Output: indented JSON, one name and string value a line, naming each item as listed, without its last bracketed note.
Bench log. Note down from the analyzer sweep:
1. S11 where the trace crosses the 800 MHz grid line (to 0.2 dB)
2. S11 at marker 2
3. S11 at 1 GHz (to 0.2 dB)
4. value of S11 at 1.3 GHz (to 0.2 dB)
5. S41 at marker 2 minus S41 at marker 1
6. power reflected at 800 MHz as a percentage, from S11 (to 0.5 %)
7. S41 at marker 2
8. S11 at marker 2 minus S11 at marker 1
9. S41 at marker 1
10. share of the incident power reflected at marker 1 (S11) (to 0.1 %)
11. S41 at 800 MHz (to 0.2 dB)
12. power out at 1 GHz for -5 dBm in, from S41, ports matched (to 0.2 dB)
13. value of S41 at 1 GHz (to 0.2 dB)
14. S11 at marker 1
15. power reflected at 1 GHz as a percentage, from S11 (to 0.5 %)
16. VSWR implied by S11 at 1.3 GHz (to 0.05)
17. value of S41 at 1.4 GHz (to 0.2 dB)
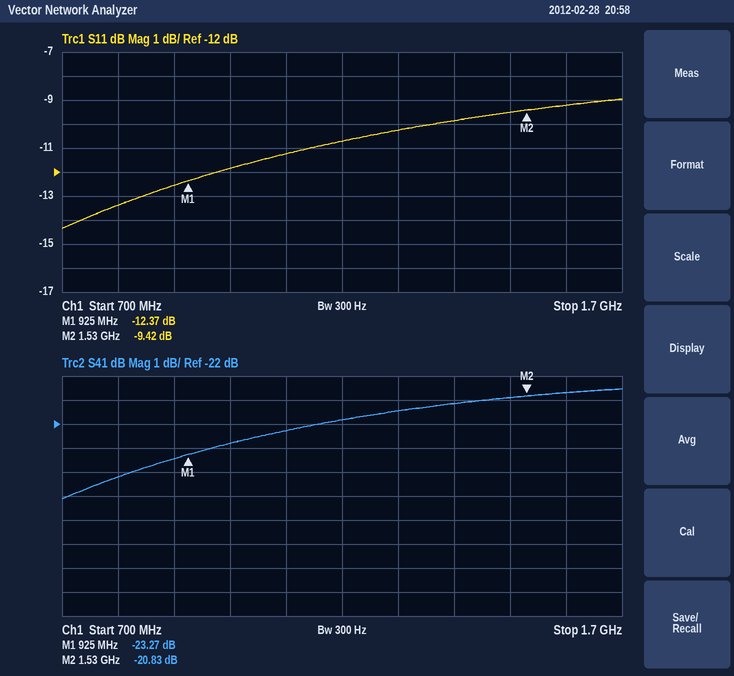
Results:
{
  "S11 where the trace crosses the 800 MHz grid line": "-13.4 dB",
  "S11 at marker 2": "-9.42 dB",
  "S11 at 1 GHz": "-11.8 dB",
  "value of S11 at 1.3 GHz": "-10.2 dB",
  "S41 at marker 2 minus S41 at marker 1": "2.44 dB",
  "power reflected at 800 MHz as a percentage, from S11": "4.5 %",
  "S41 at marker 2": "-20.83 dB",
  "S11 at marker 2 minus S11 at marker 1": "2.95 dB",
  "S41 at marker 1": "-23.27 dB",
  "share of the incident power reflected at marker 1 (S11)": "5.8 %",
  "S41 at 800 MHz": "-24.2 dB",
  "power out at 1 GHz for -5 dBm in, from S41, ports matched": "-27.8 dBm",
  "value of S41 at 1 GHz": "-22.8 dB",
  "S11 at marker 1": "-12.37 dB",
  "power reflected at 1 GHz as a percentage, from S11": "6.5 %",
  "VSWR implied by S11 at 1.3 GHz": "1.90",
  "value of S41 at 1.4 GHz": "-21.2 dB"
}
